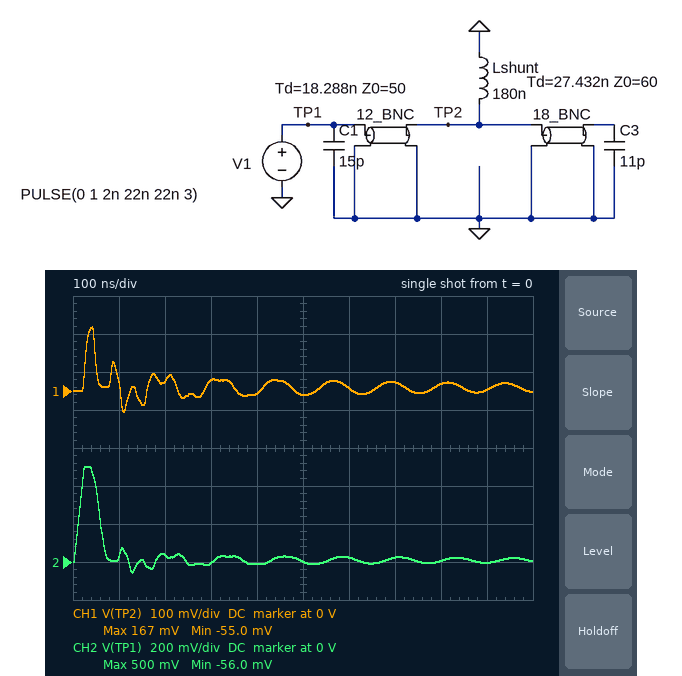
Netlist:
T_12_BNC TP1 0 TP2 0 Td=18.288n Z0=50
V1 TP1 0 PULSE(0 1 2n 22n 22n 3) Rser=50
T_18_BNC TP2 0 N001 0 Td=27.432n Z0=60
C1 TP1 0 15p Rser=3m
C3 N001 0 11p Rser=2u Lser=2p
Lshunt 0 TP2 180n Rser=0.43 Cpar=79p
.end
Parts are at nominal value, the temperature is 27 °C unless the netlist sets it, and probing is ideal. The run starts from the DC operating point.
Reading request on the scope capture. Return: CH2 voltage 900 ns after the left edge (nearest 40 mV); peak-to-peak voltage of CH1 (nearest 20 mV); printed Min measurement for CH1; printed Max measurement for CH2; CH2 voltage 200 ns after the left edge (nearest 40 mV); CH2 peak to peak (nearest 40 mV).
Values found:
0 V
220 mV
-55.0 mV
500 mV
40 mV
560 mV
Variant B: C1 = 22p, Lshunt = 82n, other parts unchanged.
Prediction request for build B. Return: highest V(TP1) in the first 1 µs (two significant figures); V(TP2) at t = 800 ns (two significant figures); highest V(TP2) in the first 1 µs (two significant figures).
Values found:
500 mV
12 mV
83 mV
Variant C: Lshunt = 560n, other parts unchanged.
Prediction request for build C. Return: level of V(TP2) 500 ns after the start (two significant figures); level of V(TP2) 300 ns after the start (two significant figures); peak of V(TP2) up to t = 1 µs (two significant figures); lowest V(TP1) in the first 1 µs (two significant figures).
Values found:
22 mV
-52 mV
340 mV
-120 mV
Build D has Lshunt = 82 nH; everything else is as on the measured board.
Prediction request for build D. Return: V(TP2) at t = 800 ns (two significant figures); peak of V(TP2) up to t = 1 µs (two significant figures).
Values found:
11 mV
83 mV
